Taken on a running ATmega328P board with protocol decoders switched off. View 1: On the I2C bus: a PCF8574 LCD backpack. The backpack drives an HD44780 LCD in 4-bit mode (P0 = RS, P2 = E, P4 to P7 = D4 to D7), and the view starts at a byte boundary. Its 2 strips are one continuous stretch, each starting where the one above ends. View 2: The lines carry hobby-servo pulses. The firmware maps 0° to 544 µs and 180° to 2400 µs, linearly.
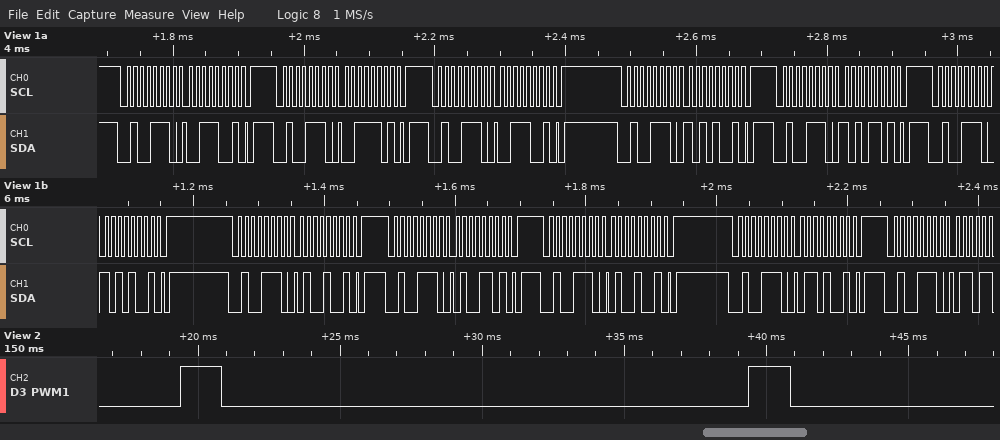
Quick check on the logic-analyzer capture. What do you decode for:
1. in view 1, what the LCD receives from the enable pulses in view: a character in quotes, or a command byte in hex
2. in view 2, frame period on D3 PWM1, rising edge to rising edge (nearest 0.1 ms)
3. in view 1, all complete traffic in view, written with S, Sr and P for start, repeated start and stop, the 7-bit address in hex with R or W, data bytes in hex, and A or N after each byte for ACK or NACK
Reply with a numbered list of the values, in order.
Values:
1. ':'
2. 20.0 ms
3. S 27W A 39 A P S 27W A 3D A P S 27W A 39 A P S 27W A A9 A P S 27W A AD A P S 27W A A9 A P S 27W A 49 A P S 27W A 4D A P S 27W A 49 A P S 27W A 69 A P S 27W A
